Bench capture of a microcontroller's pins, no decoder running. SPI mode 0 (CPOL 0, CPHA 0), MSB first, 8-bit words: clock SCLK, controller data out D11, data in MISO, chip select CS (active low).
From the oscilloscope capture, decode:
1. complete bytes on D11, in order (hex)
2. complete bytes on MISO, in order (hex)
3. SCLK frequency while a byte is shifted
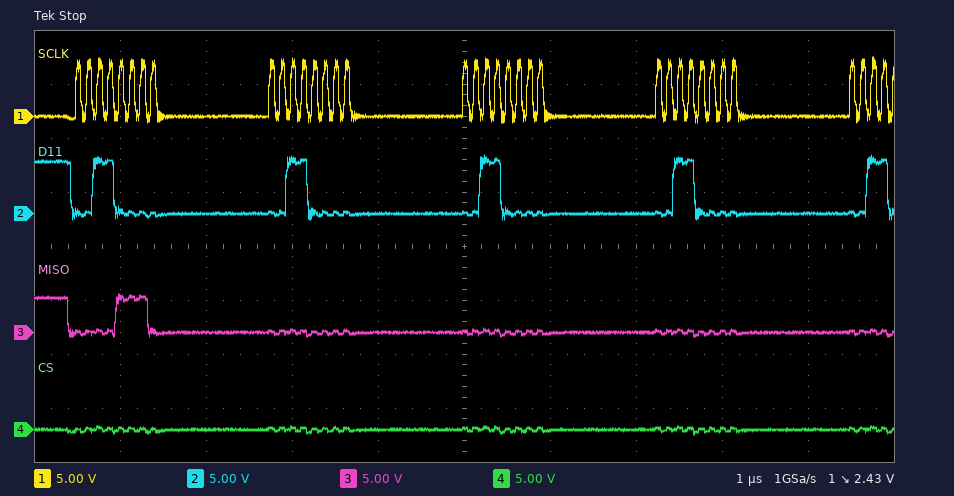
30 30 30 30
0E 00 00 00
8 MHz
